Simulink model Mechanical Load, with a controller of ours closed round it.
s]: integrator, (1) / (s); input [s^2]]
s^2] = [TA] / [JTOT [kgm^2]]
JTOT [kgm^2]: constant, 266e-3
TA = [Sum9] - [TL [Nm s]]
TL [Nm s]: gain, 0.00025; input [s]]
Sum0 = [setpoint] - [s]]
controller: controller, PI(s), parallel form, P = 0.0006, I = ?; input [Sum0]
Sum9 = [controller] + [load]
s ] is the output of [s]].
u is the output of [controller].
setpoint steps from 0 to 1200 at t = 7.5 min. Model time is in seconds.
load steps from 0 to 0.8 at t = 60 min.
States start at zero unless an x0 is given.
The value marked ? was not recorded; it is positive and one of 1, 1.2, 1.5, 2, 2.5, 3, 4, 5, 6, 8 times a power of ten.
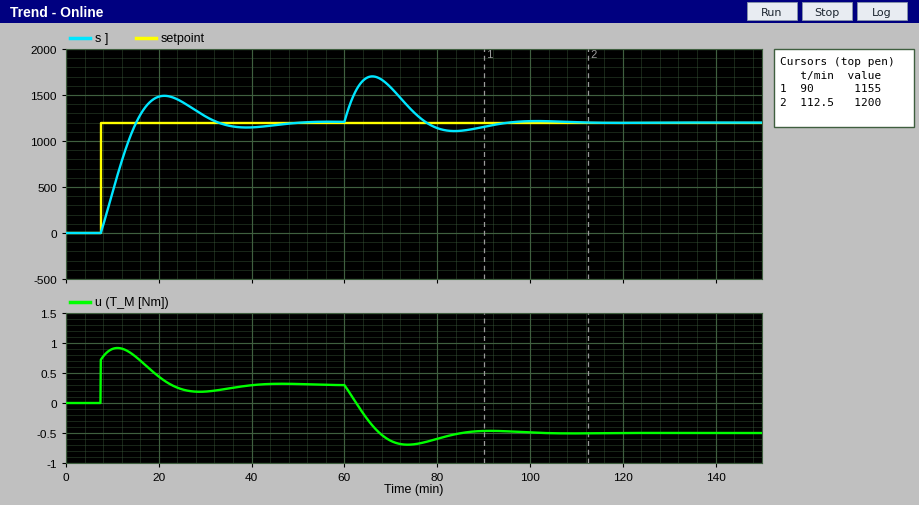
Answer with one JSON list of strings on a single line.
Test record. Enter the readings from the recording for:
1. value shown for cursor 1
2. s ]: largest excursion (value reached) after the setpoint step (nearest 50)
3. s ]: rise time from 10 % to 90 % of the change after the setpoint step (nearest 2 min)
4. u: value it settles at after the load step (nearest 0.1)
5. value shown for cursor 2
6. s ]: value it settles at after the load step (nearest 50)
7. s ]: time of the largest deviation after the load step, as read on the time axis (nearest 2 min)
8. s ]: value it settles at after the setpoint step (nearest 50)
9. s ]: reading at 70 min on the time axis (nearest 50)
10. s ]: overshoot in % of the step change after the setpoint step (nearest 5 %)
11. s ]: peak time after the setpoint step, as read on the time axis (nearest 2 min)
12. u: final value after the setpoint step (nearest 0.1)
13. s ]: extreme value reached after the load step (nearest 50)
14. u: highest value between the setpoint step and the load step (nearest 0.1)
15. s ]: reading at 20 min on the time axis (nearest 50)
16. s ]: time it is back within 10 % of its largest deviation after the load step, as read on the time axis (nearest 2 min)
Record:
["1155", "1500", "6 min", "-0.5", "1200", "1200", "66 min", "1200", "1600", "25 %", "22 min", "0.3", "1700", "0.9", "1500", "90 min"]
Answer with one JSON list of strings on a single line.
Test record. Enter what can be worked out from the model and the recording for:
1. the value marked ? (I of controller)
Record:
["3e-06"]
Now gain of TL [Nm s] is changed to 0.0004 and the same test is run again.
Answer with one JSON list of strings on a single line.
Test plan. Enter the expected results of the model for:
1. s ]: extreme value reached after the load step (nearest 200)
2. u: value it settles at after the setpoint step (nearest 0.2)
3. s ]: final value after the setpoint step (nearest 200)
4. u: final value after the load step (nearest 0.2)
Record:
["1600", "0.4", "1200", "-0.4"]
